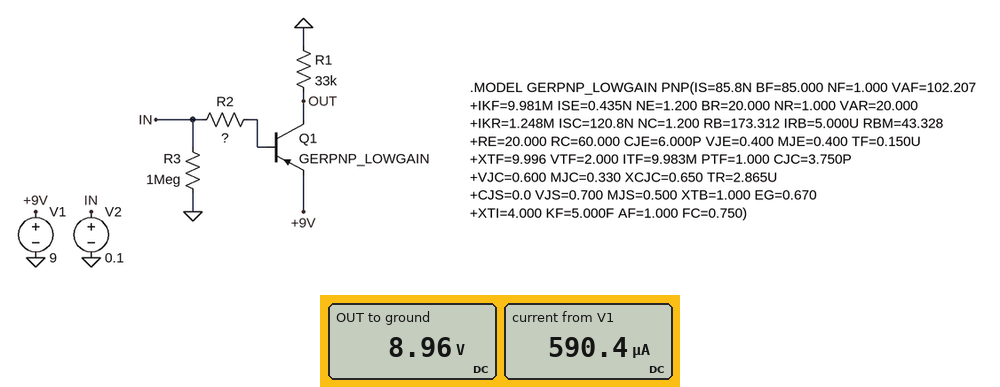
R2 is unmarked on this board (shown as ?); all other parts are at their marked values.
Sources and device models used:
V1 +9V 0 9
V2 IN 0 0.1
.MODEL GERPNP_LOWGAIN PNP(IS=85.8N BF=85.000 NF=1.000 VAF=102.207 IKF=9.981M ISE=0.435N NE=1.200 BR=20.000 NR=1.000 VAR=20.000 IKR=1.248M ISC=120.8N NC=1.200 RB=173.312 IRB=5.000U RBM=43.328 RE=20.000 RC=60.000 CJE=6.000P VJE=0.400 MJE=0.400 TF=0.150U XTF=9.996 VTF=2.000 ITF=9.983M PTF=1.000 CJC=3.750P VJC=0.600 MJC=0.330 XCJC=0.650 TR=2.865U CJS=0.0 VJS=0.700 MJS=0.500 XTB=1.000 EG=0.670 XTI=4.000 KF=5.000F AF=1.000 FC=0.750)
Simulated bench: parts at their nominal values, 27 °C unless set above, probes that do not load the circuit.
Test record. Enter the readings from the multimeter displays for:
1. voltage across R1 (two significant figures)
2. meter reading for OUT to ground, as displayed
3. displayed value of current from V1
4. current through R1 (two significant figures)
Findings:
9.0 V
8.96 V
590.4 µA
270 µA
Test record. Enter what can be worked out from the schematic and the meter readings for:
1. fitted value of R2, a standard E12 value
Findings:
27 kΩ
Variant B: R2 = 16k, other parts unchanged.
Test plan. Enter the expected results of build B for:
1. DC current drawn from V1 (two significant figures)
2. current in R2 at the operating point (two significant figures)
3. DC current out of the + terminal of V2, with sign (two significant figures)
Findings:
810 µA
540 µA
-540 µA
